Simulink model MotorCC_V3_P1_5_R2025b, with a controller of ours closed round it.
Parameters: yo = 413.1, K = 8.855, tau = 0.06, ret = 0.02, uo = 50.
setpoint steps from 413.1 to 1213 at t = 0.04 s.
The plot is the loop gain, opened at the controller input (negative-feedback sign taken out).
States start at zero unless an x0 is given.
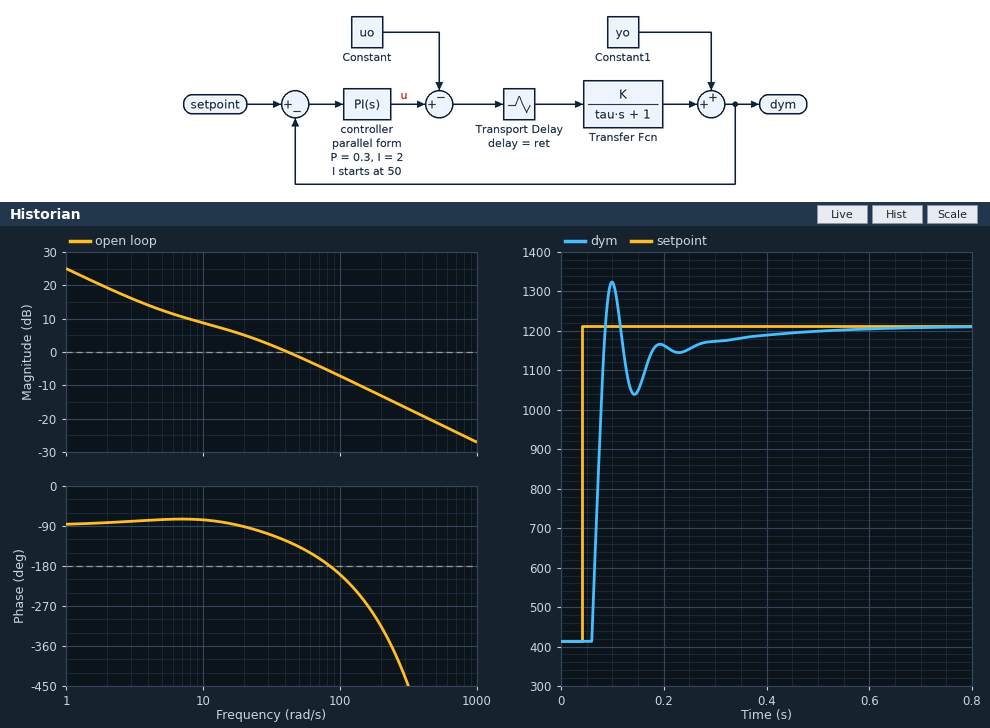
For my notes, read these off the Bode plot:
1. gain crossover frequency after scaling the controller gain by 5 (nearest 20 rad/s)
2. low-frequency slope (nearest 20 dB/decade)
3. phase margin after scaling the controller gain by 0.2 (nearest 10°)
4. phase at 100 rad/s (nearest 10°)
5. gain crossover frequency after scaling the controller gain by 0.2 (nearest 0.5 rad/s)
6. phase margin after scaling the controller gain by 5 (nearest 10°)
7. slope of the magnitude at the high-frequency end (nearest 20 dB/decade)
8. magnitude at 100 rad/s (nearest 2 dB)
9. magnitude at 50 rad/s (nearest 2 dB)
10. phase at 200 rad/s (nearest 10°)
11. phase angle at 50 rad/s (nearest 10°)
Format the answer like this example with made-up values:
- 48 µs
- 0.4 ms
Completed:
- 220 rad/s
- -20 dB/decade
- 100°
- -200°
- 4.0 rad/s
- -160°
- -20 dB/decade
- -8 dB
- -2 dB
- -320°
- -140°
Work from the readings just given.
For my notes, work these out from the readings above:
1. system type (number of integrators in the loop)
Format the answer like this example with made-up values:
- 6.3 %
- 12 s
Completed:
- 1
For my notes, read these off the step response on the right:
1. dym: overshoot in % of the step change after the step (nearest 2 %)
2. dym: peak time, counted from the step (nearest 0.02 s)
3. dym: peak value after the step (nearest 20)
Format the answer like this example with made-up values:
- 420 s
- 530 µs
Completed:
- 14 %
- 0.06 s
- 1320
